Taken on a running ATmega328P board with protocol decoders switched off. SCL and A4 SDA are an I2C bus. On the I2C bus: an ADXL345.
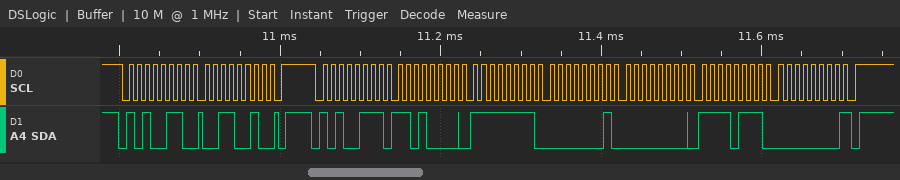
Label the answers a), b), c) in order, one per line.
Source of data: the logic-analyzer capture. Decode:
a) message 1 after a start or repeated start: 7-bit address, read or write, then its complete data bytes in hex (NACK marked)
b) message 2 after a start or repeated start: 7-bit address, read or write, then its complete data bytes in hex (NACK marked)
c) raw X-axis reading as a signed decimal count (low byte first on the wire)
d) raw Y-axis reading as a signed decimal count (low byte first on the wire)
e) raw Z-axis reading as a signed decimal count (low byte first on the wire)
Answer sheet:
a) 0x53 write: 32
b) 0x53 read: D0 FF 01 00 F7 00 NACK
c) -48
d) 1
e) 247
